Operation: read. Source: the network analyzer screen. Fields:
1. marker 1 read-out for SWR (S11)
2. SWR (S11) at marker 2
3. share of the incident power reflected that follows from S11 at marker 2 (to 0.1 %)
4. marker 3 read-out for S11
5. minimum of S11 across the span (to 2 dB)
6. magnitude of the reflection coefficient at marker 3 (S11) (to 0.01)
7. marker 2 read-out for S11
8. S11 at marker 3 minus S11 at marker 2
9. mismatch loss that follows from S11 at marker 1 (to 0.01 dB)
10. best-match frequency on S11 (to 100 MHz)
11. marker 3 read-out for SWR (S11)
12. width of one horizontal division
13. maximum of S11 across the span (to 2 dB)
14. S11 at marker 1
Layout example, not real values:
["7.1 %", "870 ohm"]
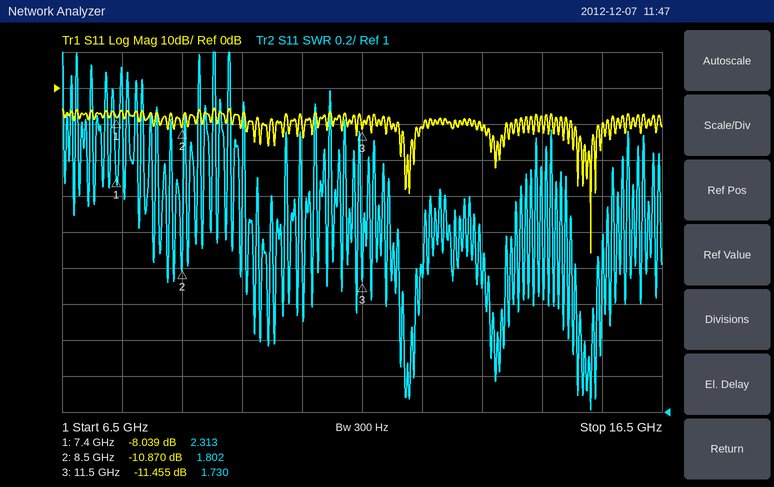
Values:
["2.313", "1.802", "8.2 %", "-11.455 dB", "-46 dB", "0.27", "-10.870 dB", "-0.585 dB", "0.74 dB", "15.3 GHz", "1.730", "1 GHz", "-6 dB", "-8.039 dB"]
